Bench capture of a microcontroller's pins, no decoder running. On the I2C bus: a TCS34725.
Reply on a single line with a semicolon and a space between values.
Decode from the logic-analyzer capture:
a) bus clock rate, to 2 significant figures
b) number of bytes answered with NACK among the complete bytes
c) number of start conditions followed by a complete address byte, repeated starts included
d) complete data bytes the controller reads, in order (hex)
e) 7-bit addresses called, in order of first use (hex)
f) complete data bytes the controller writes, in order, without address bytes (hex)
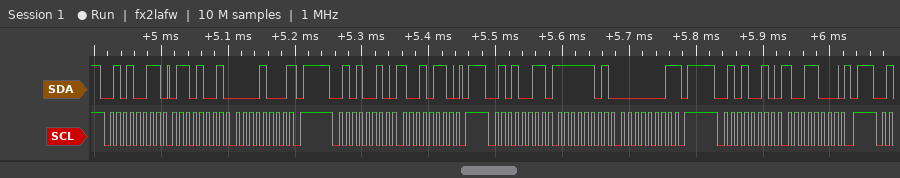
100 kHz; 2; 4; 69 08 FD 01; 0x29; 96 98
